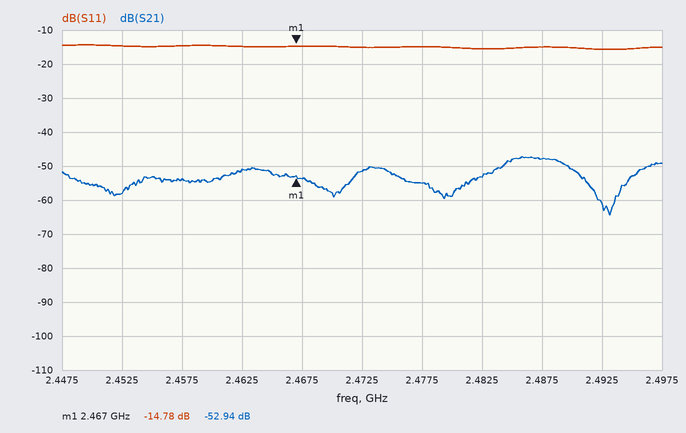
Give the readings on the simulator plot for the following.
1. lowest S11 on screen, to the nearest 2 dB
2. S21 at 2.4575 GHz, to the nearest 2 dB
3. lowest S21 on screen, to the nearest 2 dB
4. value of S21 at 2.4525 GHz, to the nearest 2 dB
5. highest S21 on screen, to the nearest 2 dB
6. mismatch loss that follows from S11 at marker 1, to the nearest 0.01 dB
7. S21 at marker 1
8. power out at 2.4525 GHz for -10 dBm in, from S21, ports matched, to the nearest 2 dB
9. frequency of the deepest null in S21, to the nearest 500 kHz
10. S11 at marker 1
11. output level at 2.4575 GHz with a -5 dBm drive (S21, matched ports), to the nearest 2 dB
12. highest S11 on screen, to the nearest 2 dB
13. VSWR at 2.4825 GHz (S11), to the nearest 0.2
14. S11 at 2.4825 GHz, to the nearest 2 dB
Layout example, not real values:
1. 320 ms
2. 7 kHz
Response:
1. -16 dB
2. -54 dB
3. -64 dB
4. -58 dB
5. -48 dB
6. 0.15 dB
7. -52.94 dB
8. -68 dBm
9. 2.4930 GHz
10. -14.78 dB
11. -58 dBm
12. -14 dB
13. 1.4
14. -16 dB
